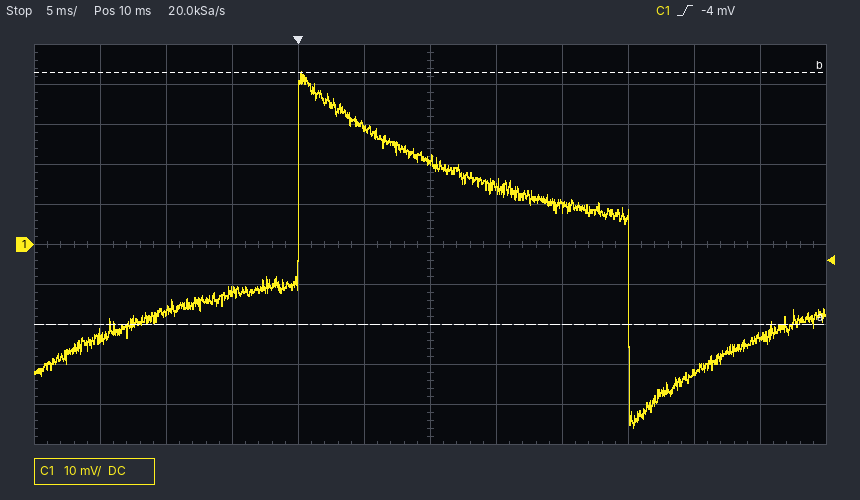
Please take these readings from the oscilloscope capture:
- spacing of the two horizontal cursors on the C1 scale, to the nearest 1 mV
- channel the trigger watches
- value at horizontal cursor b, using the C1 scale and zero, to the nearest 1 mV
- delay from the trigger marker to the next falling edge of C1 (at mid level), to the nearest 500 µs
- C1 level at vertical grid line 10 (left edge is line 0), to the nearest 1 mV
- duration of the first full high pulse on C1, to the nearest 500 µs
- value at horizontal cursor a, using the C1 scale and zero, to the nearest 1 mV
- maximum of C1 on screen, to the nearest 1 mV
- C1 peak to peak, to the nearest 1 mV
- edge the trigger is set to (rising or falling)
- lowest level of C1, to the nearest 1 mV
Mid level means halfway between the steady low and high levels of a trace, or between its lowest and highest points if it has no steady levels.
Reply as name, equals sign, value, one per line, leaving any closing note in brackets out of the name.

spacing of the two horizontal cursors on the C1 scale, to the nearest 1 mV = 63 mV
channel the trigger watches = C1
value at horizontal cursor b, using the C1 scale and zero, to the nearest 1 mV = 43 mV
delay from the trigger marker to the next falling edge of C1 (at mid level), to the nearest 500 µs = 25.0 ms
C1 level at vertical grid line 10 (left edge is line 0), to the nearest 1 mV = -32 mV
duration of the first full high pulse on C1, to the nearest 500 µs = 25.0 ms
value at horizontal cursor a, using the C1 scale and zero, to the nearest 1 mV = -20 mV
maximum of C1 on screen, to the nearest 1 mV = 43 mV
C1 peak to peak, to the nearest 1 mV = 89 mV
edge the trigger is set to = rising
lowest level of C1, to the nearest 1 mV = -46 mV
